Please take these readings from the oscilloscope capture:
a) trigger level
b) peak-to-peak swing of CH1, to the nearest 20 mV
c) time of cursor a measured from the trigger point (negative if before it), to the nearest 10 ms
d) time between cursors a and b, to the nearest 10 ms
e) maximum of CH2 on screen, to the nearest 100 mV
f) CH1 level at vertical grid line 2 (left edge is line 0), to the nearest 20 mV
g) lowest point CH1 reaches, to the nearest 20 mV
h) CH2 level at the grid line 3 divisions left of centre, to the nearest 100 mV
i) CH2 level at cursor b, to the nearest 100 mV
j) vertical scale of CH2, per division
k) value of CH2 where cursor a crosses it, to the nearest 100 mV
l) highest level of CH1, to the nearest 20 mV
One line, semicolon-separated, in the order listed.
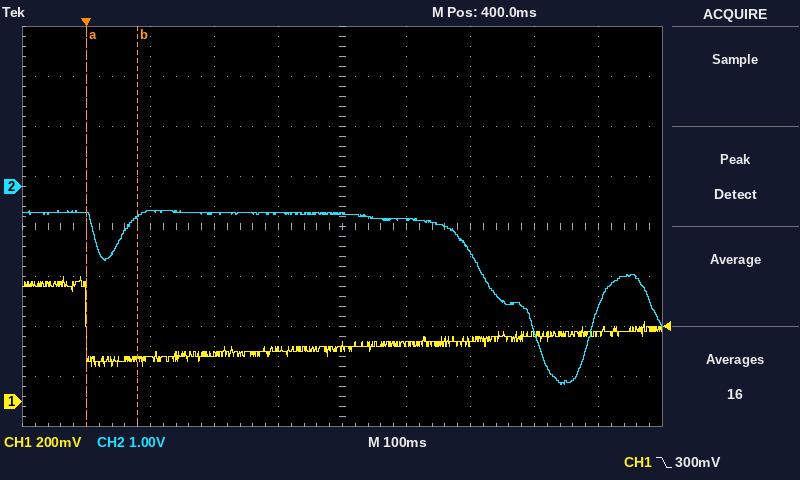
300 mV; 360 mV; 0 ms; 80 ms; -500 mV; 180 mV; 140 mV; -500 mV; -600 mV; 1 V; -600 mV; 500 mV
